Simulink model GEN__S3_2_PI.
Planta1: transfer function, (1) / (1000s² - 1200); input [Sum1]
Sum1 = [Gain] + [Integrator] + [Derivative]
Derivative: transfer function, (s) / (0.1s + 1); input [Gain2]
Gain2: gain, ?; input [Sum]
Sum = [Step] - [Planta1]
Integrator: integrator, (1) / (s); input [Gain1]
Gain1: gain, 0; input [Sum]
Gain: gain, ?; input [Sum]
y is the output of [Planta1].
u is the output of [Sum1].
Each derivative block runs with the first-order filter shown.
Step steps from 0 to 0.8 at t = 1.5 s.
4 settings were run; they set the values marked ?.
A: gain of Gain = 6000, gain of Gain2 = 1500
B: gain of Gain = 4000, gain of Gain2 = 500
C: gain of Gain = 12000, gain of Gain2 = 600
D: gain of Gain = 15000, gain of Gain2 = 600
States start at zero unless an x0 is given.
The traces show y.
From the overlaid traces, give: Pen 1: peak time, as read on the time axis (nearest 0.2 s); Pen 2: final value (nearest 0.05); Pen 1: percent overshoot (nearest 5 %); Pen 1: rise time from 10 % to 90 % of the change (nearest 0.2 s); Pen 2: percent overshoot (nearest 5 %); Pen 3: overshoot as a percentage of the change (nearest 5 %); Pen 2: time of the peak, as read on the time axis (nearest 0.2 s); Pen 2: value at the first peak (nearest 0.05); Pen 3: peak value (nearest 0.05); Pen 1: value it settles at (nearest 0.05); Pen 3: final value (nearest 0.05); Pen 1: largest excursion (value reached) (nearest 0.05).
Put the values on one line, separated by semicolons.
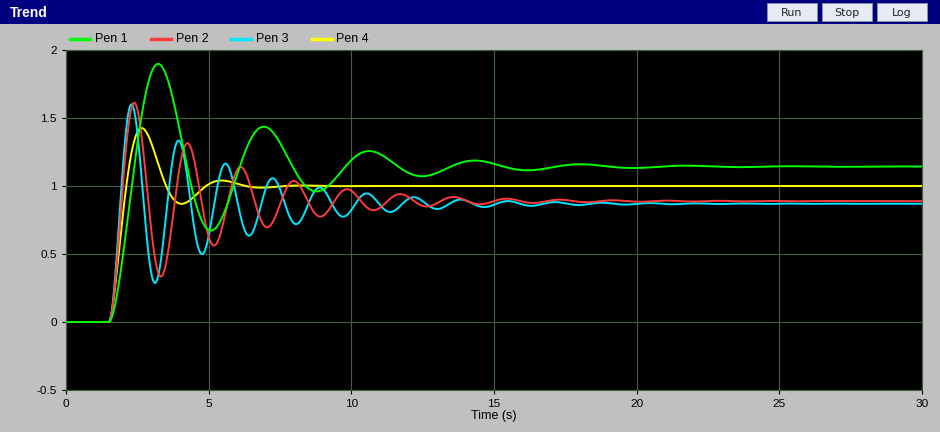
3.2 s; 0.90; 65 %; 0.6 s; 80 %; 85 %; 2.4 s; 1.60; 1.60; 1.15; 0.85; 1.90
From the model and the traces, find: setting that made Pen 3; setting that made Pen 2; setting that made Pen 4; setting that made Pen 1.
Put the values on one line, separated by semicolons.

D; C; A; B
